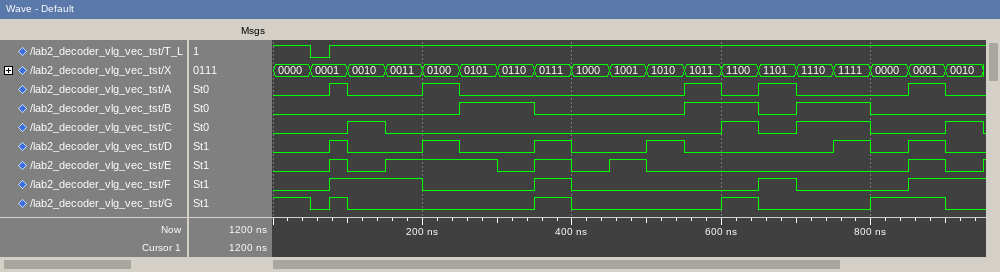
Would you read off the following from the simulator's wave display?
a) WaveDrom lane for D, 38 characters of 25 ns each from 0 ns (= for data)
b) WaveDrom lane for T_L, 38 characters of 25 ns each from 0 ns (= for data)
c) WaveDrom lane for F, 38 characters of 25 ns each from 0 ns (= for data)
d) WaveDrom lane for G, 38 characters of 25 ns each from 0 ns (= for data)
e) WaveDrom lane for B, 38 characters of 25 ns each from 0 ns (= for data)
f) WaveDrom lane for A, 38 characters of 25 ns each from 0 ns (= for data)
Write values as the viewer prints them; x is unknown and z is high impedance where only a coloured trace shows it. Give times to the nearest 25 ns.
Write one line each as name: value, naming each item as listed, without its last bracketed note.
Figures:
WaveDrom lane for D, 38 characters of 25 ns each from 0 ns: {name: 'D', wave: '0..10...1.0...1.0...1.0.......1.0.1.0.'}
WaveDrom lane for T_L, 38 characters of 25 ns each from 0 ns: {name: 'T_L', wave: '1.01..................................'}
WaveDrom lane for F, 38 characters of 25 ns each from 0 ns: {name: 'F', wave: '0..1....0.....1.0.........1.0.....1...'}
WaveDrom lane for G, 38 characters of 25 ns each from 0 ns: {name: 'G', wave: '1.010.........1.0.......1.0.....1...0.'}
WaveDrom lane for B, 38 characters of 25 ns each from 0 ns: {name: 'B', wave: '0.........1...0.......1...0.1...0.....'}
WaveDrom lane for A, 38 characters of 25 ns each from 0 ns: {name: 'A', wave: '0..10...1.0...........1.0.1.0.....1.0.'}
